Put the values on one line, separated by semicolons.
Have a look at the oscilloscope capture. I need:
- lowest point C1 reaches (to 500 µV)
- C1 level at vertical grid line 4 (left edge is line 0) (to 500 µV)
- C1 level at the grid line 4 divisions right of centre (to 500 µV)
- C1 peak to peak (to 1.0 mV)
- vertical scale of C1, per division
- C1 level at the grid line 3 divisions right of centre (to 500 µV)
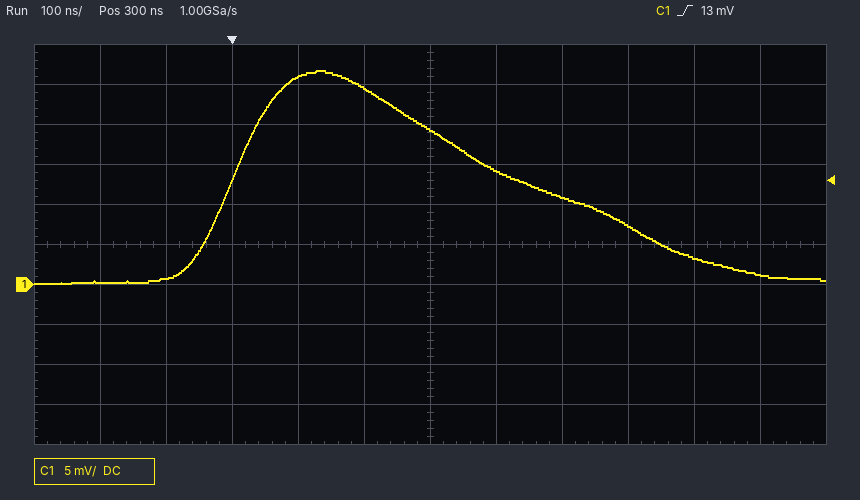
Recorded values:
0.0 mV; 26.0 mV; 3.5 mV; 27.0 mV; 5 mV; 7.5 mV
